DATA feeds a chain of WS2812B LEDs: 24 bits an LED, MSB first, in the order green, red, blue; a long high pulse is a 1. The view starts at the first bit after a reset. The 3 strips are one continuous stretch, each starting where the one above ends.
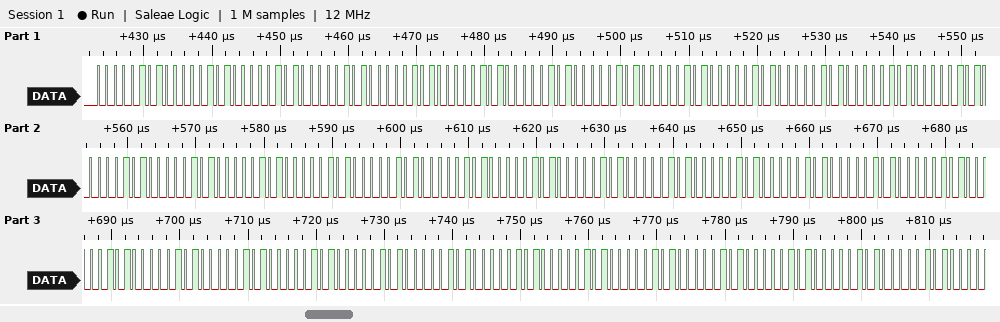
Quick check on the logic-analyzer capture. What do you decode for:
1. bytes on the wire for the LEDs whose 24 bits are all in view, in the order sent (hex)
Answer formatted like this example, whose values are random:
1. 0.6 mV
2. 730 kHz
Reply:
1. 05 05 05 05 05 05 05 05 05 05 05 05 05 05 05 05 05 05 05 05 05 05 05 05 05 05 05 05 05 05 05 05 05 05 05 05 05 05 05
